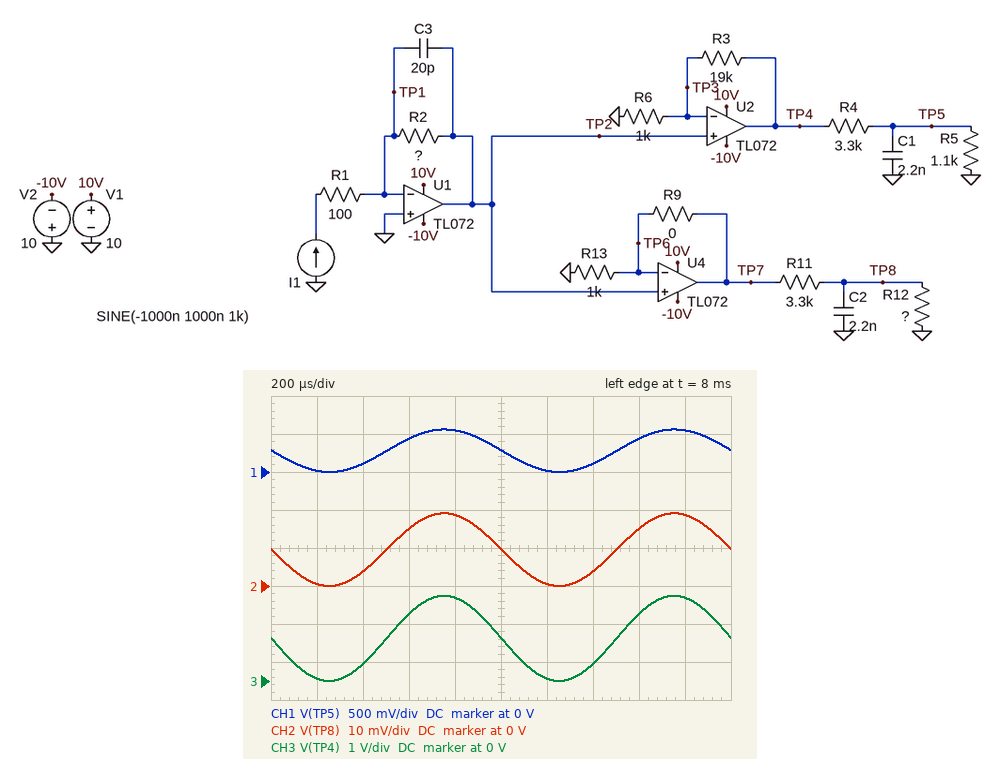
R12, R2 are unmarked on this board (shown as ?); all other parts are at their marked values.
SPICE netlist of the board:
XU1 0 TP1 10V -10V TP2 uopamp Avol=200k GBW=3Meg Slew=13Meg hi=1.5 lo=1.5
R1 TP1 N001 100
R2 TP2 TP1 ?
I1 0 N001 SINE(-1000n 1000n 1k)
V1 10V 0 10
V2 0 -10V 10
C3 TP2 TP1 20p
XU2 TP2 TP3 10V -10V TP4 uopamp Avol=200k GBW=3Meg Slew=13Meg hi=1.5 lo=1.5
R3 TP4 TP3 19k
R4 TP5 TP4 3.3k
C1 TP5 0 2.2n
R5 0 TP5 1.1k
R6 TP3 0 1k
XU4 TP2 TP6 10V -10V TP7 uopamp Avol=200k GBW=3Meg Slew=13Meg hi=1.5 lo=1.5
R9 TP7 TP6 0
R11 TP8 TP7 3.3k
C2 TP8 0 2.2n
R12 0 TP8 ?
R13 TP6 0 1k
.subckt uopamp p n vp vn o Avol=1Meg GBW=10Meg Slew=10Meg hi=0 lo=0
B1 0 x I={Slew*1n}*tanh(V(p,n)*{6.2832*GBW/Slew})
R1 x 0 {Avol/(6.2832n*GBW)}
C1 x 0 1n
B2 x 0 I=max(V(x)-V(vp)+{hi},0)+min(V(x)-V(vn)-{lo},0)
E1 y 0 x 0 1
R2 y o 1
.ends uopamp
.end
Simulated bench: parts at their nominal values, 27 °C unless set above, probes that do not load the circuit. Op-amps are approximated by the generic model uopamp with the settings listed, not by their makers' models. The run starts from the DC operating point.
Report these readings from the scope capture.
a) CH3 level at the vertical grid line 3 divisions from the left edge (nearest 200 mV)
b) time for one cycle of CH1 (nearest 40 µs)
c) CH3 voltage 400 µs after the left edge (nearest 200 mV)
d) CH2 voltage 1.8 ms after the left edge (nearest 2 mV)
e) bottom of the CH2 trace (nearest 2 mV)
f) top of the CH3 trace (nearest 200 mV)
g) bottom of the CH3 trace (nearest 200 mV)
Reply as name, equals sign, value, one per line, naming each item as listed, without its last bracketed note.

CH3 level at the vertical grid line 3 divisions from the left edge = 1.8 V
time for one cycle of CH1 = 1.00 ms
CH3 voltage 400 µs after the left edge = 400 mV
CH2 voltage 1.8 ms after the left edge = 18 mV
bottom of the CH2 trace = 0 V
top of the CH3 trace = 2.2 V
bottom of the CH3 trace = 0 V
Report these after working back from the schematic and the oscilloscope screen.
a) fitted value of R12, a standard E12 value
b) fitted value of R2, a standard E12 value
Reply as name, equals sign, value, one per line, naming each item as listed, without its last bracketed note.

fitted value of R12, a standard E12 value = 680 Ω
fitted value of R2, a standard E12 value = 56 kΩ
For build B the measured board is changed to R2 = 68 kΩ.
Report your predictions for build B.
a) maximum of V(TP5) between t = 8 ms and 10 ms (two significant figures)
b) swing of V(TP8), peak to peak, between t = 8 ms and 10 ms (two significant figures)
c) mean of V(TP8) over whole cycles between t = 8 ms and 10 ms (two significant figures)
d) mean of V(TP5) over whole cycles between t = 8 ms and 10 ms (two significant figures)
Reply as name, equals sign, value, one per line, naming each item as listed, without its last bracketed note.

maximum of V(TP5) between t = 8 ms and 10 ms = 680 mV
swing of V(TP8), peak to peak, between t = 8 ms and 10 ms = 23 mV
mean of V(TP8) over whole cycles between t = 8 ms and 10 ms = 12 mV
mean of V(TP5) over whole cycles between t = 8 ms and 10 ms = 340 mV
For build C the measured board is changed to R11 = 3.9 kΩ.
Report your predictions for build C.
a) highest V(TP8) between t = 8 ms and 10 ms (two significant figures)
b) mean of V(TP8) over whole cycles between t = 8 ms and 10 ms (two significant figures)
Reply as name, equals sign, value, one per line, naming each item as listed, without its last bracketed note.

highest V(TP8) between t = 8 ms and 10 ms = 17 mV
mean of V(TP8) over whole cycles between t = 8 ms and 10 ms = 8.3 mV
